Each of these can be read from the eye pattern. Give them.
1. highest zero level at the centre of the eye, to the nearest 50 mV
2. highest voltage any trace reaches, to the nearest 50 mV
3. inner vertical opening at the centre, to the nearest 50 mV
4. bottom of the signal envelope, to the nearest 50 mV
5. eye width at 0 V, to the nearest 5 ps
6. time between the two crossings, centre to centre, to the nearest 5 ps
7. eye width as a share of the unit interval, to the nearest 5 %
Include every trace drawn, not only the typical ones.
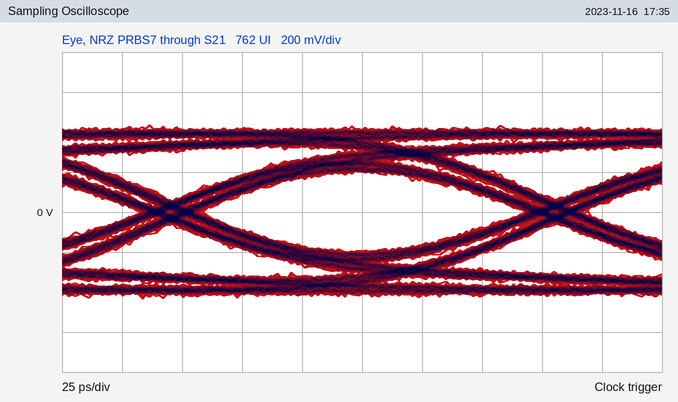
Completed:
-200 mV
450 mV
400 mV
-450 mV
135 ps
160 ps
85 %
